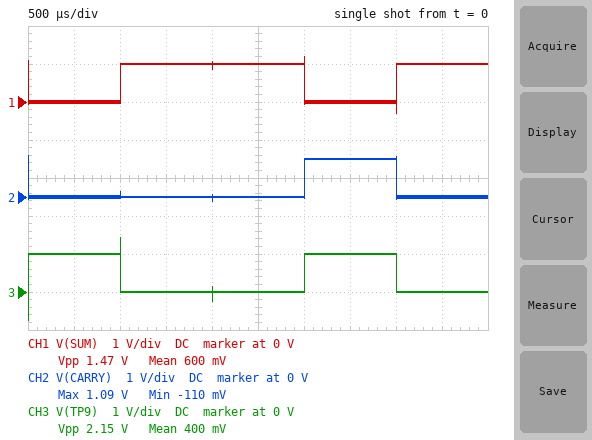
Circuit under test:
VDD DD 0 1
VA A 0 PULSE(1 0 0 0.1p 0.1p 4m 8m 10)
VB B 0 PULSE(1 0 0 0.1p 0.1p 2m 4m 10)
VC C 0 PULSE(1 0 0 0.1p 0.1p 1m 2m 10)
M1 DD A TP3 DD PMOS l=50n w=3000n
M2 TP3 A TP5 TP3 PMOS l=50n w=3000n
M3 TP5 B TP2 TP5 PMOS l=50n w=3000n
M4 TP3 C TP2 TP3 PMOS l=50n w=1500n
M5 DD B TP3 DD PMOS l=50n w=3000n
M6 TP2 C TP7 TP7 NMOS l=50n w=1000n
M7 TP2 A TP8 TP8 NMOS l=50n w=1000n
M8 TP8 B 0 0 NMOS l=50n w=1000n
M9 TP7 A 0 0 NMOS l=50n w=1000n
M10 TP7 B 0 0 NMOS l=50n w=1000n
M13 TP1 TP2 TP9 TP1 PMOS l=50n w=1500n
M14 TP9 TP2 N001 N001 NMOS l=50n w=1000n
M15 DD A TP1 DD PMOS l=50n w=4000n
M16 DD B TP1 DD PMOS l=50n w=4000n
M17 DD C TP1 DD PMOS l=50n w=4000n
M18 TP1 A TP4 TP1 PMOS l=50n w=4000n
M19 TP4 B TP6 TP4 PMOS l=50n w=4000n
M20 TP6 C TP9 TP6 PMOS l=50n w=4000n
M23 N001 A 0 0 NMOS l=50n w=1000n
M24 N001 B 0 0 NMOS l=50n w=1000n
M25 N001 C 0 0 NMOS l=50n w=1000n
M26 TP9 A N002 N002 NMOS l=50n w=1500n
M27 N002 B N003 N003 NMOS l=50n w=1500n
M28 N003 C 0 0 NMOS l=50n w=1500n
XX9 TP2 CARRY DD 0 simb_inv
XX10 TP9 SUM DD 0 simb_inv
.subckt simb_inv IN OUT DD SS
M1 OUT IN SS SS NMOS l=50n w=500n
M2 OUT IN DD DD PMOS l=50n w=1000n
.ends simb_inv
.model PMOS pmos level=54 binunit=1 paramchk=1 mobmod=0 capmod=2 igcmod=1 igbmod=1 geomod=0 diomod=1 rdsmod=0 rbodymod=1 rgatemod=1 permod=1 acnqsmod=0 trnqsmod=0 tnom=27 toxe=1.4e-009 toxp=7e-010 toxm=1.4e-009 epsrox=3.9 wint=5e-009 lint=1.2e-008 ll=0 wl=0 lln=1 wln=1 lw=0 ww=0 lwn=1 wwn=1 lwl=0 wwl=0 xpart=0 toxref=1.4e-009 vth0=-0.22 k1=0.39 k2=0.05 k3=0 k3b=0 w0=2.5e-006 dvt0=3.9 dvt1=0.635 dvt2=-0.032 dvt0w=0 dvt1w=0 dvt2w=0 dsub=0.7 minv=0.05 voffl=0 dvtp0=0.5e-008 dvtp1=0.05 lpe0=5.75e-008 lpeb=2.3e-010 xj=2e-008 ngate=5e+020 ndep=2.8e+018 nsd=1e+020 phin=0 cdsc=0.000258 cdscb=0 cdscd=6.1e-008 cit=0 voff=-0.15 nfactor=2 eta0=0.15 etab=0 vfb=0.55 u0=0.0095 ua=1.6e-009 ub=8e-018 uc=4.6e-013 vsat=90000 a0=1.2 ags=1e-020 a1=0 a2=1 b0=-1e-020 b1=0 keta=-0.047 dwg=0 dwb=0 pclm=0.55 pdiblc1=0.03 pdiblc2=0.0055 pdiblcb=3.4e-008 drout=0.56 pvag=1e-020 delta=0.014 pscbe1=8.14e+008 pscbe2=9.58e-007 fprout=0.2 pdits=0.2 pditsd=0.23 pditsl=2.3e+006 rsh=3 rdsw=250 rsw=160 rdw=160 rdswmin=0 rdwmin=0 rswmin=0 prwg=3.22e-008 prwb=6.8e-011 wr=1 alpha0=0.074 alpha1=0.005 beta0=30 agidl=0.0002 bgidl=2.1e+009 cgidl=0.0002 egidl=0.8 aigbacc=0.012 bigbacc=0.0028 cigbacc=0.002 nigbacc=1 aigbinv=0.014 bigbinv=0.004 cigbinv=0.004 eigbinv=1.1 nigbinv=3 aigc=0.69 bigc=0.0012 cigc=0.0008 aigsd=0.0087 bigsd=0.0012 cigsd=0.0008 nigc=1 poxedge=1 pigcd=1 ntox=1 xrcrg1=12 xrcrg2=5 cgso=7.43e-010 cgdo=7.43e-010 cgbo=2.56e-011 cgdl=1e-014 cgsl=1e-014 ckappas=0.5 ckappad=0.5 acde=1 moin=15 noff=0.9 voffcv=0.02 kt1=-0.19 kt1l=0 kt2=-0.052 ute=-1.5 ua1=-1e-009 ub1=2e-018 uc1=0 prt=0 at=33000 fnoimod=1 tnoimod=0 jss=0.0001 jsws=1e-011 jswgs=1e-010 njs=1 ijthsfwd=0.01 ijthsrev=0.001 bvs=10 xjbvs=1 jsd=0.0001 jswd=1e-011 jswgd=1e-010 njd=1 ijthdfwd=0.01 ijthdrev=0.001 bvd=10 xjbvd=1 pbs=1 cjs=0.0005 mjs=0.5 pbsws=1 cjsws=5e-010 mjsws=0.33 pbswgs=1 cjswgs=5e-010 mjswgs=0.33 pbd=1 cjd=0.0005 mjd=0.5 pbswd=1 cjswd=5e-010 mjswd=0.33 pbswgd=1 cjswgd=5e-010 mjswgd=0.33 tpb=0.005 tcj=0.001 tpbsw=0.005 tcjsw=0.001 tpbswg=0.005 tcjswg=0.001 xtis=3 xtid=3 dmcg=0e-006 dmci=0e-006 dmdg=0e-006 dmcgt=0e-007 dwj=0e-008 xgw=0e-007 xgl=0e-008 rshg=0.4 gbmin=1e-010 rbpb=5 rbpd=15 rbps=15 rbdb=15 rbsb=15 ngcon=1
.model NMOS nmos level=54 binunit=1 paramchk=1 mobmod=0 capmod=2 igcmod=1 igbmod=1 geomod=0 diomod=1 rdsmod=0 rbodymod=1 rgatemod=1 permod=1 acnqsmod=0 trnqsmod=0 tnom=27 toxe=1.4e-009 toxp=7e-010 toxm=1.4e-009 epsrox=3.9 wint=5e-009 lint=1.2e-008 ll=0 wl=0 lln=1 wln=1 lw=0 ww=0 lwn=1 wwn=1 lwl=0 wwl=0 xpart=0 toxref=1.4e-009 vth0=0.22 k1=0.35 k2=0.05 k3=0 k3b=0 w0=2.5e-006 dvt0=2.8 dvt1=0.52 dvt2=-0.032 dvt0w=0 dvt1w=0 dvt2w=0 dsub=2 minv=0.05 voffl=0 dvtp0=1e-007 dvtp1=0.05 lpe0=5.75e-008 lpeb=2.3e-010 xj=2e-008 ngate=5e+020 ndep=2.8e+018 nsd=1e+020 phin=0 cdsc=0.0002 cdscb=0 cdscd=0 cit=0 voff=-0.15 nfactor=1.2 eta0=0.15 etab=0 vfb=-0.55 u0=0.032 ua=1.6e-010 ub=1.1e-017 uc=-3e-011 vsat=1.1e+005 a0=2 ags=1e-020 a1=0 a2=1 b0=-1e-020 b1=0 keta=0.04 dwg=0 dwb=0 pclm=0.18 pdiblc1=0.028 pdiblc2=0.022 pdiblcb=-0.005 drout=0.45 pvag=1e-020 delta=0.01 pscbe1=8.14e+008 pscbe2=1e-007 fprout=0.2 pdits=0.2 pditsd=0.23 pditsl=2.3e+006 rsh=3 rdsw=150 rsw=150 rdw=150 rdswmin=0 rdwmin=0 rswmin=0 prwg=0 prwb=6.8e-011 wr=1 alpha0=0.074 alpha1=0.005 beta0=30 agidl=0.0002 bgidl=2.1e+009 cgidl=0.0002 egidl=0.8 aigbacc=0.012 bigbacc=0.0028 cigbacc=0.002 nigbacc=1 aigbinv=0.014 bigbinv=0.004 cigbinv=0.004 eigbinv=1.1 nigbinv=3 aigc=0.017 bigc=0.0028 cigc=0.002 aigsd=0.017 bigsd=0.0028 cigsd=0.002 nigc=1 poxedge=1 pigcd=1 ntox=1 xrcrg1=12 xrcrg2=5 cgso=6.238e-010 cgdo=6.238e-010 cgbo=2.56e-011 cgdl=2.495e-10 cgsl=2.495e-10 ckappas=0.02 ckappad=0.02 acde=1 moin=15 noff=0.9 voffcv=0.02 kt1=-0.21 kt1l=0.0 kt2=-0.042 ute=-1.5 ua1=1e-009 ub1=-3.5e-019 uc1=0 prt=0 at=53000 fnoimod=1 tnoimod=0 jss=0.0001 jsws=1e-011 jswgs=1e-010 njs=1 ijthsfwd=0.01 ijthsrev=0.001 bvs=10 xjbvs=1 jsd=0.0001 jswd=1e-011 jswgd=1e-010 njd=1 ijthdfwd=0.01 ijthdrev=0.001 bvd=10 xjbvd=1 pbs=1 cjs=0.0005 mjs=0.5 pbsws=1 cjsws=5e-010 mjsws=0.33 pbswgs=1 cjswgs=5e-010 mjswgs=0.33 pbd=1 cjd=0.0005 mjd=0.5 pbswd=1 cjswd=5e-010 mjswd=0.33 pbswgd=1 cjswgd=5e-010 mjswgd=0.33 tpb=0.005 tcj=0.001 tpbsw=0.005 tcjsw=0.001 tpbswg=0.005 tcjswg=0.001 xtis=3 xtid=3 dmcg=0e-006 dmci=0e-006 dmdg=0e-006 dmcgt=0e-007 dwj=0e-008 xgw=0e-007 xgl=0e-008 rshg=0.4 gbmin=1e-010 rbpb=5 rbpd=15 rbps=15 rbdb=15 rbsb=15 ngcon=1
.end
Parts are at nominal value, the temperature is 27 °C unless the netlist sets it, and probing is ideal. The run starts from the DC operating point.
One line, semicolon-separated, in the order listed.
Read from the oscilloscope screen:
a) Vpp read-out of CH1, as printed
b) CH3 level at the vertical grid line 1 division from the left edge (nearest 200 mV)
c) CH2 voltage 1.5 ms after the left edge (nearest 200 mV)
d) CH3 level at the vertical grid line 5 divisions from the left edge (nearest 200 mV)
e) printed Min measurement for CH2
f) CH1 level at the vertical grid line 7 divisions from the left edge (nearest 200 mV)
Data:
1.47 V; 1.0 V; 0 V; 0 V; -110 mV; 0 V
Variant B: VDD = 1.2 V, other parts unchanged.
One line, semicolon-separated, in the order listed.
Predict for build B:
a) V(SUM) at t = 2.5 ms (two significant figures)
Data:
1.2 V
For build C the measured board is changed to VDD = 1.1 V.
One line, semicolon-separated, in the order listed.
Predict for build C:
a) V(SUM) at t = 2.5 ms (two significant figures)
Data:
1.1 V
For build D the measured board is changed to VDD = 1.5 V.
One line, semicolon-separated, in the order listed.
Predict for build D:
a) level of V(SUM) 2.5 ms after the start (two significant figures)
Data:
1.5 V
